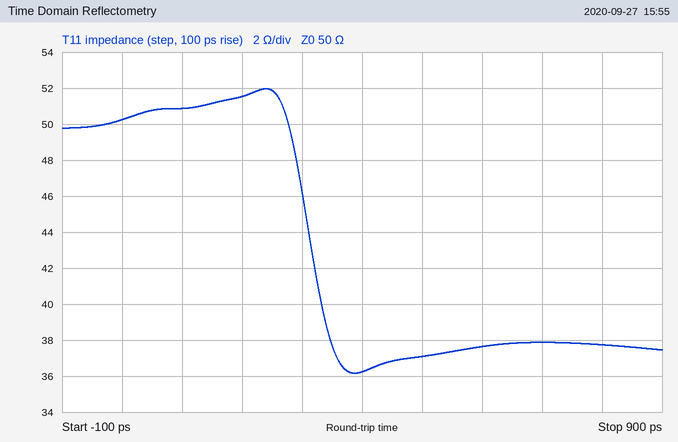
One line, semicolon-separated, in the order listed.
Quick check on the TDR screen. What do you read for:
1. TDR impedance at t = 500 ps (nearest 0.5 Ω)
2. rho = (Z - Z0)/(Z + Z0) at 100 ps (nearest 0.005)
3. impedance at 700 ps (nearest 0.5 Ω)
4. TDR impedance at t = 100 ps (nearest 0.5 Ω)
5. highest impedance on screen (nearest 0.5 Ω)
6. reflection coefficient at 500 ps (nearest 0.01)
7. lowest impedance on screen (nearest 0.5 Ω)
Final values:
37.0 Ω; +0.010; 38.0 Ω; 51.0 Ω; 52.0 Ω; -0.15; 36.0 Ω
